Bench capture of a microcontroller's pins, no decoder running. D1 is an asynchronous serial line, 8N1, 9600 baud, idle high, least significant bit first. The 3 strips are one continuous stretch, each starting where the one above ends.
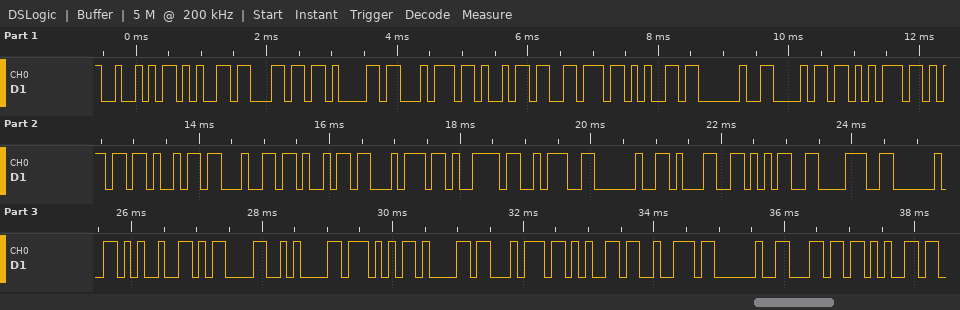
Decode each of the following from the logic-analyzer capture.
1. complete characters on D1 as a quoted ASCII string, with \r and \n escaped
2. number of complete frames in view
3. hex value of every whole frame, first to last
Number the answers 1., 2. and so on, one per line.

1. "Relative humidity: 158 %\r\nWater le"
2. 34
3. 52 65 6C 61 74 69 76 65 20 68 75 6D 69 64 69 74 79 3A 20 31 35 38 20 25 0D 0A 57 61 74 65 72 20 6C 65
